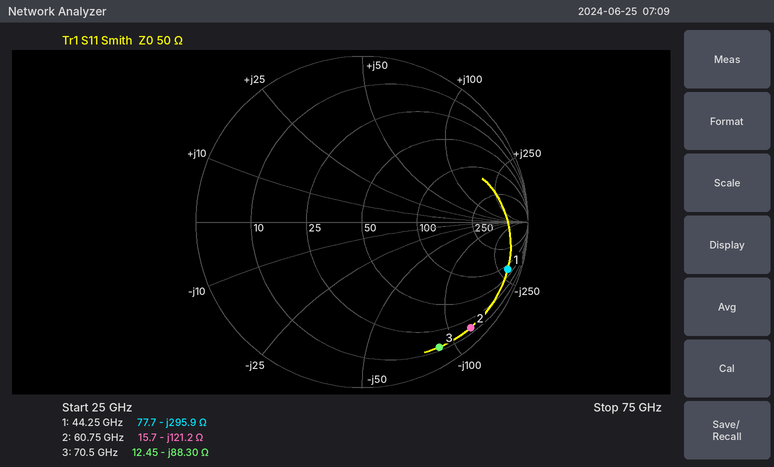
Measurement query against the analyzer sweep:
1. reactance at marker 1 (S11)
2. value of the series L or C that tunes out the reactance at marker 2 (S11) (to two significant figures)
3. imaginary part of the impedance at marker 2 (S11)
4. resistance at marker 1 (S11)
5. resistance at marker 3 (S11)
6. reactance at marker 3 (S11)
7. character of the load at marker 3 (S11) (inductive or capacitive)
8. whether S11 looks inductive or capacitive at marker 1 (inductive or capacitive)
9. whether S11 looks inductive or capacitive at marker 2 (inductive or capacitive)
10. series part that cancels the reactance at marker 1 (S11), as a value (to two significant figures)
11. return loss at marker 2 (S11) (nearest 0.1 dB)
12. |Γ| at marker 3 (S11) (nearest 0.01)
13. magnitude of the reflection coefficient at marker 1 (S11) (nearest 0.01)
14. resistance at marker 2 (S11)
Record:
-295.9 Ω
320 pH
-121.2 Ω
77.7 Ω
12.45 Ω
-88.30 Ω
capacitive
capacitive
capacitive
1.1 nH
0.8 dB
0.89
0.92
15.7 Ω
